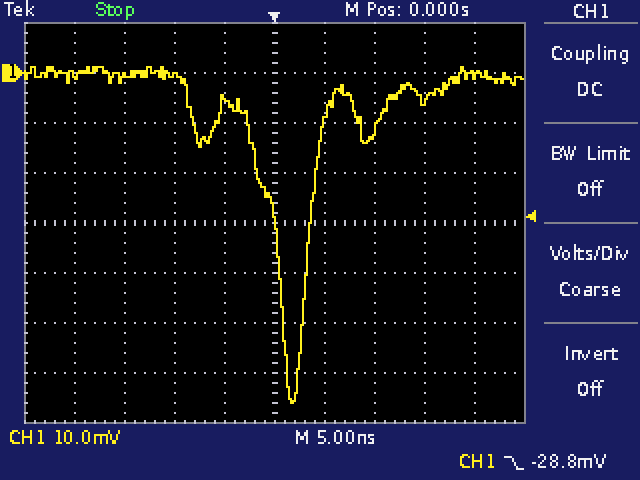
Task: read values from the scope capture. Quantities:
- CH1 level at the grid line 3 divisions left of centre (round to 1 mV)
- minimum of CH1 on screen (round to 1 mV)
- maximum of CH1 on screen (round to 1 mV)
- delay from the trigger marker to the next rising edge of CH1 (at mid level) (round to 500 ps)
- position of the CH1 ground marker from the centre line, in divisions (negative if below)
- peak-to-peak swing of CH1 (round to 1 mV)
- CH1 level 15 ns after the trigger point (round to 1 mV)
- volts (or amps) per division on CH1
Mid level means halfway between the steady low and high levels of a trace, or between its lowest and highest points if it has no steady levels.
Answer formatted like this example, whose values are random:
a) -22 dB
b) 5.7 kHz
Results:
a) -1 mV
b) -66 mV
c) 1 mV
d) 3.5 ns
e) +3.0 div
f) 67 mV
g) -5 mV
h) 10 mV
